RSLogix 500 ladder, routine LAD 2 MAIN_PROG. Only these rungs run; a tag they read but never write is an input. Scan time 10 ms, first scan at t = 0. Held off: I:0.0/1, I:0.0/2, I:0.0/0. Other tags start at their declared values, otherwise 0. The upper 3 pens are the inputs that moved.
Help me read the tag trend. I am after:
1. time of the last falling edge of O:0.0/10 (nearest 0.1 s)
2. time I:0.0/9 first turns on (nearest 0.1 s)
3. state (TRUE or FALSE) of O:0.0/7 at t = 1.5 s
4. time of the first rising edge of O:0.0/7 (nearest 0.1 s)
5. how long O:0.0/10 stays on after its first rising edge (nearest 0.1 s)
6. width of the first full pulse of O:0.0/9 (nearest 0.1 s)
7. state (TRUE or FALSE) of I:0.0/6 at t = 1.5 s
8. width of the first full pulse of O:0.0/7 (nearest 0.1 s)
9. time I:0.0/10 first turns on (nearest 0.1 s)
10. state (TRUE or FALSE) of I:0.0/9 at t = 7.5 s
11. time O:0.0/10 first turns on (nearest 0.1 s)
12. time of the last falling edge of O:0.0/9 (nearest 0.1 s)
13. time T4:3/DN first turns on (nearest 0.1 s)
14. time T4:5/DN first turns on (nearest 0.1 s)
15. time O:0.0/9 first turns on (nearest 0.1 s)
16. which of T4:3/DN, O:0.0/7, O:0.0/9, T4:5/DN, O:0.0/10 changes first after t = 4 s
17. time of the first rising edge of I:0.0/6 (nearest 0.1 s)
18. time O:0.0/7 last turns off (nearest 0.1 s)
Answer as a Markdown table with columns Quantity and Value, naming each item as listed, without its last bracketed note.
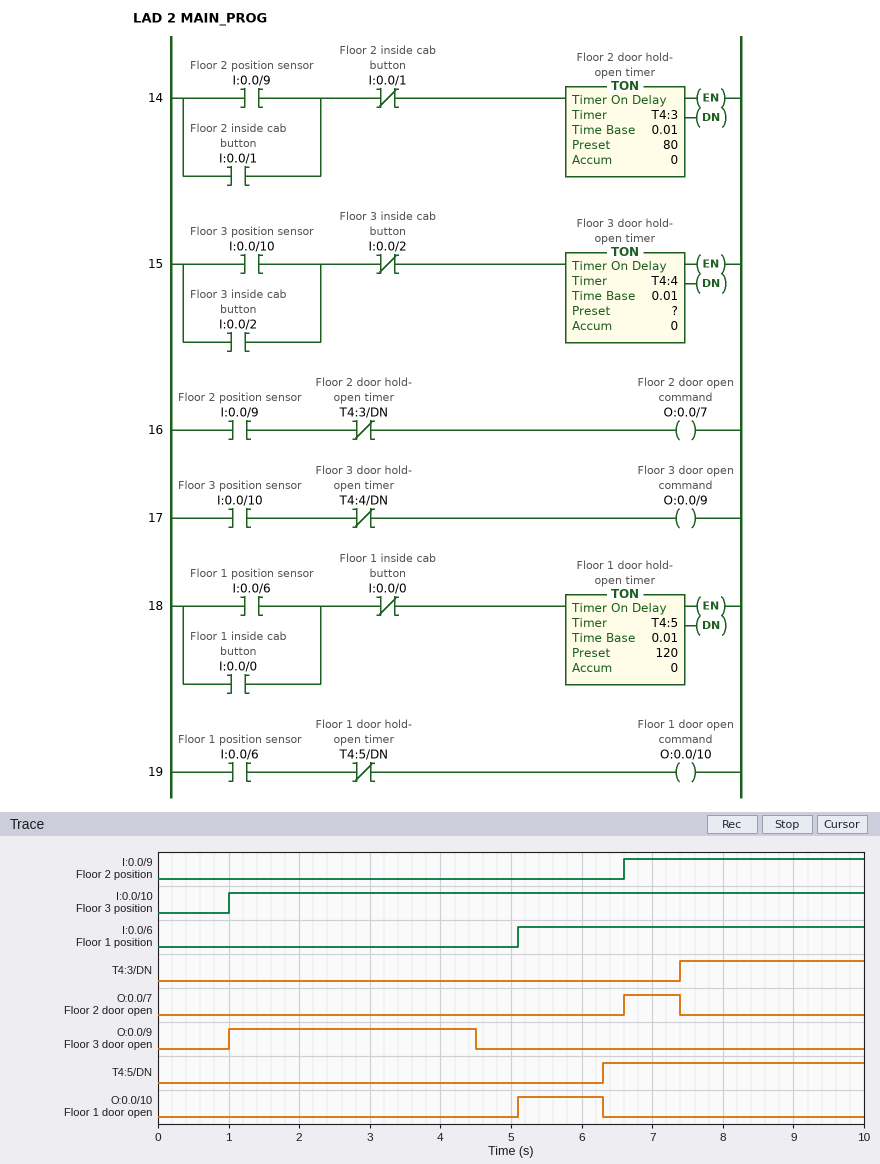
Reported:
| Quantity | Value |
|---|---|
| time of the last falling edge of O:0.0/10 | 6.3 s |
| time I:0.0/9 first turns on | 6.6 s |
| state (TRUE or FALSE) of O:0.0/7 at t = 1.5 s | FALSE |
| time of the first rising edge of O:0.0/7 | 6.6 s |
| how long O:0.0/10 stays on after its first rising edge | 1.2 s |
| width of the first full pulse of O:0.0/9 | 3.5 s |
| state (TRUE or FALSE) of I:0.0/6 at t = 1.5 s | FALSE |
| width of the first full pulse of O:0.0/7 | 0.8 s |
| time I:0.0/10 first turns on | 1.0 s |
| state (TRUE or FALSE) of I:0.0/9 at t = 7.5 s | TRUE |
| time O:0.0/10 first turns on | 5.1 s |
| time of the last falling edge of O:0.0/9 | 4.5 s |
| time T4:3/DN first turns on | 7.4 s |
| time T4:5/DN first turns on | 6.3 s |
| time O:0.0/9 first turns on | 1.0 s |
| which of T4:3/DN, O:0.0/7, O:0.0/9, T4:5/DN, O:0.0/10 changes first after t = 4 s | O:0.0/9 |
| time of the first rising edge of I:0.0/6 | 5.1 s |
| time O:0.0/7 last turns off | 7.4 s |
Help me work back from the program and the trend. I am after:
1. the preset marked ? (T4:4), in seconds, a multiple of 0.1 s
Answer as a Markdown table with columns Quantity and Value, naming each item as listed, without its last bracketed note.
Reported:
| Quantity | Value |
|---|---|
| the preset marked ? (T4:4), in seconds, a multiple of 0.1 s | 3.5 s |
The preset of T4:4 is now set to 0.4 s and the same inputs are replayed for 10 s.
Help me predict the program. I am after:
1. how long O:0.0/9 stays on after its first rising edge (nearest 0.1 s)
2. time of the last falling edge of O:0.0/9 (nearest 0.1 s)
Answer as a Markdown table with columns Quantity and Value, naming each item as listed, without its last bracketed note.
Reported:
| Quantity | Value |
|---|---|
| how long O:0.0/9 stays on after its first rising edge | 0.4 s |
| time of the last falling edge of O:0.0/9 | 1.4 s |
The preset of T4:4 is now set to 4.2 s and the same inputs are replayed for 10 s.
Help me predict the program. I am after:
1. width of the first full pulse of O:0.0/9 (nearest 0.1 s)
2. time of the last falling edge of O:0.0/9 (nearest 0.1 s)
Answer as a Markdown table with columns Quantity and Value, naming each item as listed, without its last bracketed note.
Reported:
| Quantity | Value |
|---|---|
| width of the first full pulse of O:0.0/9 | 4.2 s |
| time of the last falling edge of O:0.0/9 | 5.2 s |
